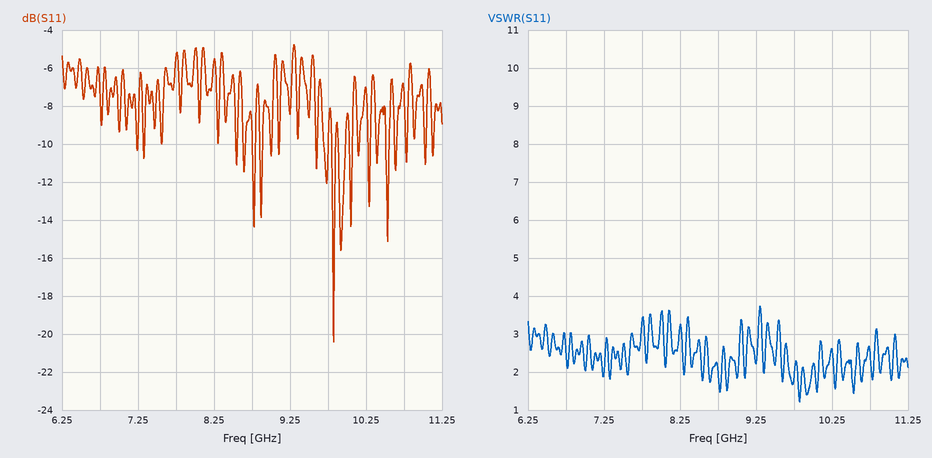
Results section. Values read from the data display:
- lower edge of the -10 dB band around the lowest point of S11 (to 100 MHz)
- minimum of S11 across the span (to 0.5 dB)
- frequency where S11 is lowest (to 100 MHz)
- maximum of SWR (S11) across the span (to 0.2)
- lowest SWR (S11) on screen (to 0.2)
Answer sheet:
9.8 GHz
-20.5 dB
9.8 GHz
3.8
1.2
